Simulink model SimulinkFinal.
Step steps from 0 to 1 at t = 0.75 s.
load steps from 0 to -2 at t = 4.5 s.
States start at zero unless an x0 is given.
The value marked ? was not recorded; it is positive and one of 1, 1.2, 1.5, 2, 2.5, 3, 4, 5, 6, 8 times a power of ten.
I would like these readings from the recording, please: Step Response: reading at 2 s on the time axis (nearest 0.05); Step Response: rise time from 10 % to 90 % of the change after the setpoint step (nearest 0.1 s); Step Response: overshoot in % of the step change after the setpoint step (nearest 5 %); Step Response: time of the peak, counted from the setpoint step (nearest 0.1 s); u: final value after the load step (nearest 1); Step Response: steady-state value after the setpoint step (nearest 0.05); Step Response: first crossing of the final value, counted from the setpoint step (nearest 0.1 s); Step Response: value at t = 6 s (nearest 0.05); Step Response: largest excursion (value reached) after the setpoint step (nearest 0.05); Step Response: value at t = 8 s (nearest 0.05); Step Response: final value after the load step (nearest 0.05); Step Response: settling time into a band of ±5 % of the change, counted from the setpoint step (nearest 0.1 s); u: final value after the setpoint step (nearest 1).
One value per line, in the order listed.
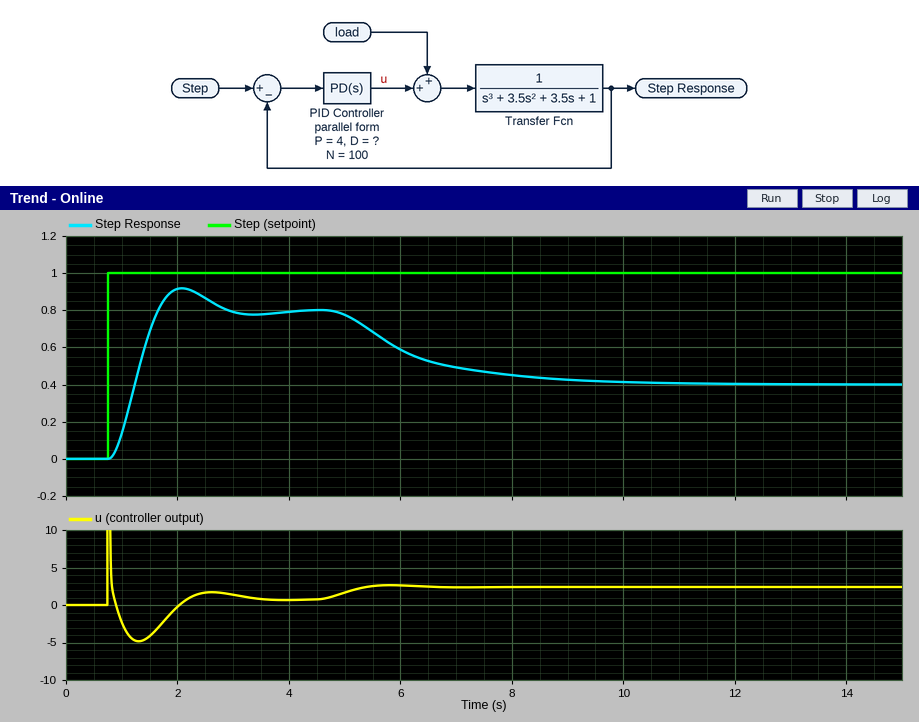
0.90
0.6 s
15 %
1.3 s
2
0.80
0.9 s
0.60
0.90
0.45
0.40
1.9 s
1
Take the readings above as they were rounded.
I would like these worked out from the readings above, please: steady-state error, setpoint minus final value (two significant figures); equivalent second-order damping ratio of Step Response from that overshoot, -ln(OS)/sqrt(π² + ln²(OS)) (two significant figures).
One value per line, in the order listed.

0.20
0.52
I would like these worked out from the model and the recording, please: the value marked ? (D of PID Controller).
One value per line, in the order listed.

6
